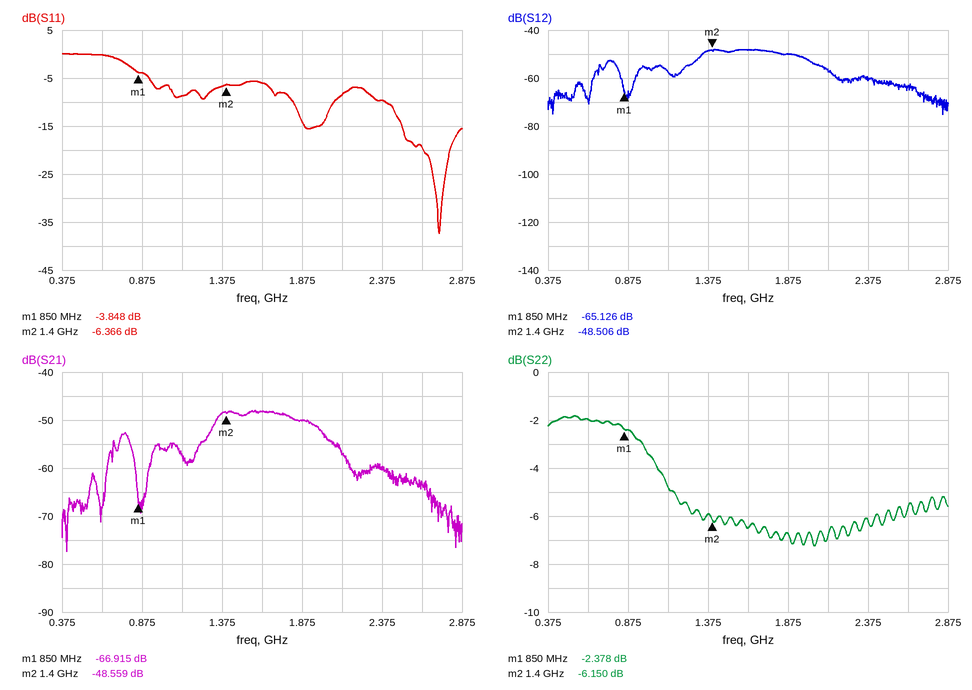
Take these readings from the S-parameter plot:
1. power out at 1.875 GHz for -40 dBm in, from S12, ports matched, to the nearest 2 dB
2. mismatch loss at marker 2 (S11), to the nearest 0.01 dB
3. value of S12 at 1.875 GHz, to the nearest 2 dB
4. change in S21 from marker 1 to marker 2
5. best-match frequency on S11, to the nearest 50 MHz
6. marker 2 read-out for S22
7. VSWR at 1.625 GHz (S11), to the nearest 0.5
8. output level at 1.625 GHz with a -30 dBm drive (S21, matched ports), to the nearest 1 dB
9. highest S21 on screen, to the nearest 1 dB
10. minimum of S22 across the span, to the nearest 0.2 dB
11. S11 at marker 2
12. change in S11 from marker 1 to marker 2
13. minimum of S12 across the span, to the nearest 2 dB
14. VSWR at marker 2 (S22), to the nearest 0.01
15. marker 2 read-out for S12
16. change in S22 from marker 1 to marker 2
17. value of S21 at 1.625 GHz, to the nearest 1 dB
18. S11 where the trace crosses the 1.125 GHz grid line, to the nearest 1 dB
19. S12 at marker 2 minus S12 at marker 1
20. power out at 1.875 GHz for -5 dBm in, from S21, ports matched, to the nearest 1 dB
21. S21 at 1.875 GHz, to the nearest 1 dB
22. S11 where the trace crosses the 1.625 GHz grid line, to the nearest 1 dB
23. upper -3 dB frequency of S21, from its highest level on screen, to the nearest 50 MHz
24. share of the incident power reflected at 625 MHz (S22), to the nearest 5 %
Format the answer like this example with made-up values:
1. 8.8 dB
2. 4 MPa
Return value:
1. -90 dBm
2. 1.14 dB
3. -50 dB
4. 18.356 dB
5. 2.75 GHz
6. -6.150 dB
7. 3.0
8. -78 dBm
9. -48 dB
10. -7.2 dB
11. -6.366 dB
12. -2.518 dB
13. -76 dB
14. 2.94
15. -48.506 dB
16. -3.772 dB
17. -48 dB
18. -9 dB
19. 16.620 dB
20. -55 dBm
21. -50 dB
22. -6 dB
23. 1.95 GHz
24. 65 %
